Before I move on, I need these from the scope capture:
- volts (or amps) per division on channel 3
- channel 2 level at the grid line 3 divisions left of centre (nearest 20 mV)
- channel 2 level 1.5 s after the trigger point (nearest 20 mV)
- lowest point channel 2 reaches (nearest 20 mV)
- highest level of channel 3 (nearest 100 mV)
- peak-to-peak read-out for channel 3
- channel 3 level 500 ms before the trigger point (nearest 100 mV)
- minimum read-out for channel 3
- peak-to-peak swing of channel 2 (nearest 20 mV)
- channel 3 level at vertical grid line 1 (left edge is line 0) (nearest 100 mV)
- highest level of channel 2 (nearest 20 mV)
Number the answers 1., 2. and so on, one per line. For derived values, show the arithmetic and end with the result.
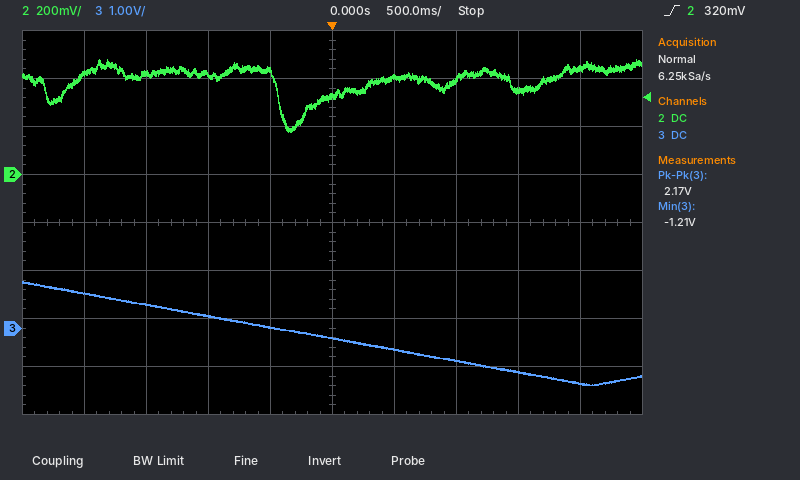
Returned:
1. 1 V
2. 420 mV
3. 340 mV
4. 180 mV
5. 1.0 V
6. 2.17 V
7. 0.0 V
8. -1.21 V
9. 480 mV − (180 mV) = 300 mV
10. 700 mV
11. 480 mV
